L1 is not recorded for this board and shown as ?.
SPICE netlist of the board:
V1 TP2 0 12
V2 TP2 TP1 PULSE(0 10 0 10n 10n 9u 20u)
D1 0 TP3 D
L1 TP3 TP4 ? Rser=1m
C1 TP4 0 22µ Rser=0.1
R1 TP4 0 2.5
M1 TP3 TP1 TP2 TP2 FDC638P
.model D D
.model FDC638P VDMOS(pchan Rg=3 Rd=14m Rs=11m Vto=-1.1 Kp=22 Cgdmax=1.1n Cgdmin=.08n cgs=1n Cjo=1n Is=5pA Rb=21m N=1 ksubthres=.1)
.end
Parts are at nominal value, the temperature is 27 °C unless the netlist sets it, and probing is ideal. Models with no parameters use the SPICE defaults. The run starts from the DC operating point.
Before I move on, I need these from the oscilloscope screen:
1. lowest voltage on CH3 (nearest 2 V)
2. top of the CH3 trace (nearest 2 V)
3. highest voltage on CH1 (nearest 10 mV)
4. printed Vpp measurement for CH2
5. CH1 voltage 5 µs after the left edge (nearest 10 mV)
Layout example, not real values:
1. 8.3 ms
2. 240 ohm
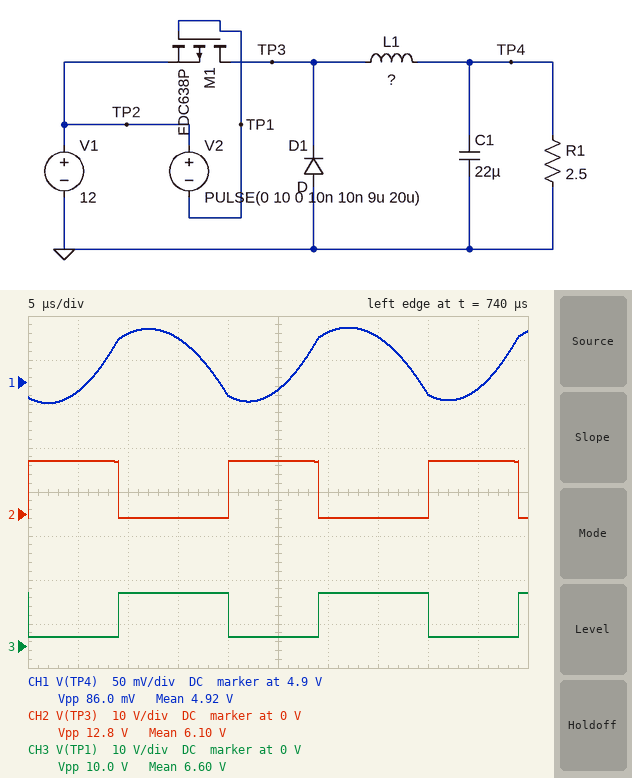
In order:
1. 2 V
2. 12 V
3. 4.96 V
4. 12.8 V
5. 4.89 V
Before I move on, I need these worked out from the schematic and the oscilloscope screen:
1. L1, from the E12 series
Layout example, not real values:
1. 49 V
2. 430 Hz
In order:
1. 100 µH
